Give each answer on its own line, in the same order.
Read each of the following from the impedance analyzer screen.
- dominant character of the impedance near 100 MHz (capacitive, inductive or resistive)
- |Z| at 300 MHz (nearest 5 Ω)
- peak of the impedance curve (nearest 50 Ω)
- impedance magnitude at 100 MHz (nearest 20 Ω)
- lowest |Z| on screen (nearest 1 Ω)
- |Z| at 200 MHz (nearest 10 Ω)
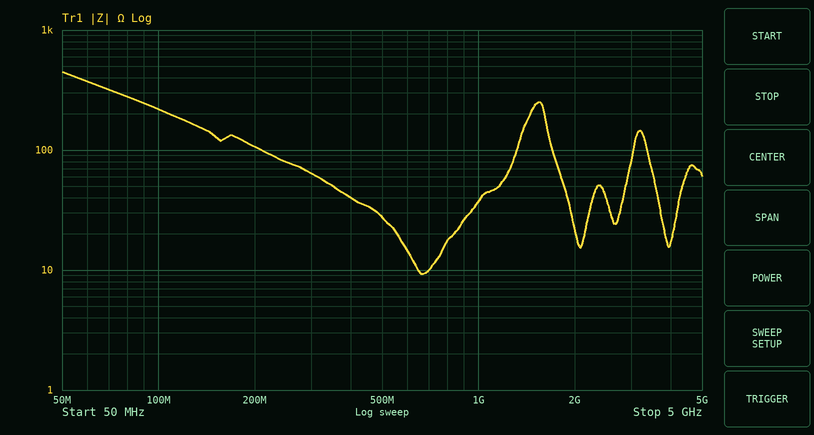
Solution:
capacitive
65 Ω
450 Ω
220 Ω
9 Ω
110 Ω
